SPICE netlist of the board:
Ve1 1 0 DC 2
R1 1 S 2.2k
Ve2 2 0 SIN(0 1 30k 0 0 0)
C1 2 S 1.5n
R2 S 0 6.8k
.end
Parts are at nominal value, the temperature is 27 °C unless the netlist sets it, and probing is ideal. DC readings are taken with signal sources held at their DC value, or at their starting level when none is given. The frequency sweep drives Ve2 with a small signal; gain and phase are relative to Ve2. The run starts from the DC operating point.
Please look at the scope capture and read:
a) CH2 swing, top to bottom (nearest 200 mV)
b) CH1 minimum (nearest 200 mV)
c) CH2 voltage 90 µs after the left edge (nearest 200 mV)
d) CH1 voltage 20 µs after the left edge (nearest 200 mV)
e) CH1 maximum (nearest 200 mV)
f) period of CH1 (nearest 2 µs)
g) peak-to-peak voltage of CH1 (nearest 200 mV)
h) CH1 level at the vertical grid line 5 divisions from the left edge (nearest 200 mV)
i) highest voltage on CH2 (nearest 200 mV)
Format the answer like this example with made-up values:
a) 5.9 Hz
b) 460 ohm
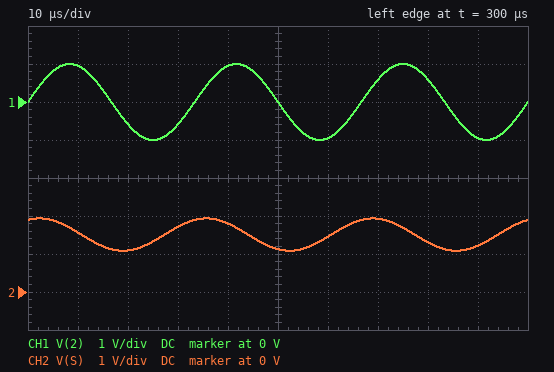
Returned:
a) 800 mV
b) -1.0 V
c) 1.2 V
d) -600 mV
e) 1.0 V
f) 34 µs
g) 2.0 V
h) 0 V
i) 2.0 V
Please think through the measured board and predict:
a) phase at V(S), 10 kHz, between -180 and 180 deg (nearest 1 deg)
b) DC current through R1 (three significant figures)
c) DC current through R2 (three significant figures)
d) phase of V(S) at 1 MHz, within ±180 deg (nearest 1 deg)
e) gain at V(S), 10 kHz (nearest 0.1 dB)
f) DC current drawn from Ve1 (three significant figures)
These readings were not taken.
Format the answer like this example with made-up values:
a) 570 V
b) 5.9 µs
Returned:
a) 81 deg
b) 222 µA
c) 222 µA
d) 4 deg
e) -16.2 dB
f) 222 µA
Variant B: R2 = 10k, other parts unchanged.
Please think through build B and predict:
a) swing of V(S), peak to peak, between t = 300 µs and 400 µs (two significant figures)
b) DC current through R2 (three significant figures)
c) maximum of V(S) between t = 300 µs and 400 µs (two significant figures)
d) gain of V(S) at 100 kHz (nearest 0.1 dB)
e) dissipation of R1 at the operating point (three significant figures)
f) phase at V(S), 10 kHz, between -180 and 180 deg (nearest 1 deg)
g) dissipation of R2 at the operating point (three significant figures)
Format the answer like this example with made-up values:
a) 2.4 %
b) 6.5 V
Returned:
a) 910 mV
b) 164 µA
c) 2.1 V
d) -1.3 dB
e) 59.1 µW
f) 80 deg
g) 269 µW
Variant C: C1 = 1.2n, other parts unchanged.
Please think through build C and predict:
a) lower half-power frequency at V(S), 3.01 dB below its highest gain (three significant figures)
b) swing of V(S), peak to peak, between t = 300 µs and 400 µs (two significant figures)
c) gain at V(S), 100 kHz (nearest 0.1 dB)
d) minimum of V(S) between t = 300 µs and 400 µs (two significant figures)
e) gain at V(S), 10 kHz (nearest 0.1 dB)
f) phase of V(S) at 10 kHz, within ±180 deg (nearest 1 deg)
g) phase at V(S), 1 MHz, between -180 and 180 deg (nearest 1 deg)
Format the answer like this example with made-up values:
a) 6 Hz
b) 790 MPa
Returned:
a) 79.8 kHz
b) 700 mV
c) -2.1 dB
d) 1.2 V
e) -18.1 dB
f) 83 deg
g) 5 deg
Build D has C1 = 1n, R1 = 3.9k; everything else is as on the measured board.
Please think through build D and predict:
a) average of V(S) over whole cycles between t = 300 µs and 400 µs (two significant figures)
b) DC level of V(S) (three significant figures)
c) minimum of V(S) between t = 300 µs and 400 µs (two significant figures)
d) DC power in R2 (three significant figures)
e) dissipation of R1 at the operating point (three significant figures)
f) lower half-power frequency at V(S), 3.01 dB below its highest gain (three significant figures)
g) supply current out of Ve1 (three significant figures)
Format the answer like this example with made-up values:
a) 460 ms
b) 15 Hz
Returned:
a) 1.3 V
b) 1.27 V
c) 850 mV
d) 238 µW
e) 136 µW
f) 64.2 kHz
g) 187 µA
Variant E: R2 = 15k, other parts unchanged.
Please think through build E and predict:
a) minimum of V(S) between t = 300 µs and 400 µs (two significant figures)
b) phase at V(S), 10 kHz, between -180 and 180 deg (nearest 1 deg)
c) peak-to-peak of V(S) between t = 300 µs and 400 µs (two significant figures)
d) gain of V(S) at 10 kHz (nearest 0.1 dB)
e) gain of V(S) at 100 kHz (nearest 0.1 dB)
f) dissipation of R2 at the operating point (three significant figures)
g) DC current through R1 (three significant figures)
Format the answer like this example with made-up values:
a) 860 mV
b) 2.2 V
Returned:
a) 1.3 V
b) 80 deg
c) 950 mV
d) -15.0 dB
e) -1.2 dB
f) 203 µW
g) 116 µA
